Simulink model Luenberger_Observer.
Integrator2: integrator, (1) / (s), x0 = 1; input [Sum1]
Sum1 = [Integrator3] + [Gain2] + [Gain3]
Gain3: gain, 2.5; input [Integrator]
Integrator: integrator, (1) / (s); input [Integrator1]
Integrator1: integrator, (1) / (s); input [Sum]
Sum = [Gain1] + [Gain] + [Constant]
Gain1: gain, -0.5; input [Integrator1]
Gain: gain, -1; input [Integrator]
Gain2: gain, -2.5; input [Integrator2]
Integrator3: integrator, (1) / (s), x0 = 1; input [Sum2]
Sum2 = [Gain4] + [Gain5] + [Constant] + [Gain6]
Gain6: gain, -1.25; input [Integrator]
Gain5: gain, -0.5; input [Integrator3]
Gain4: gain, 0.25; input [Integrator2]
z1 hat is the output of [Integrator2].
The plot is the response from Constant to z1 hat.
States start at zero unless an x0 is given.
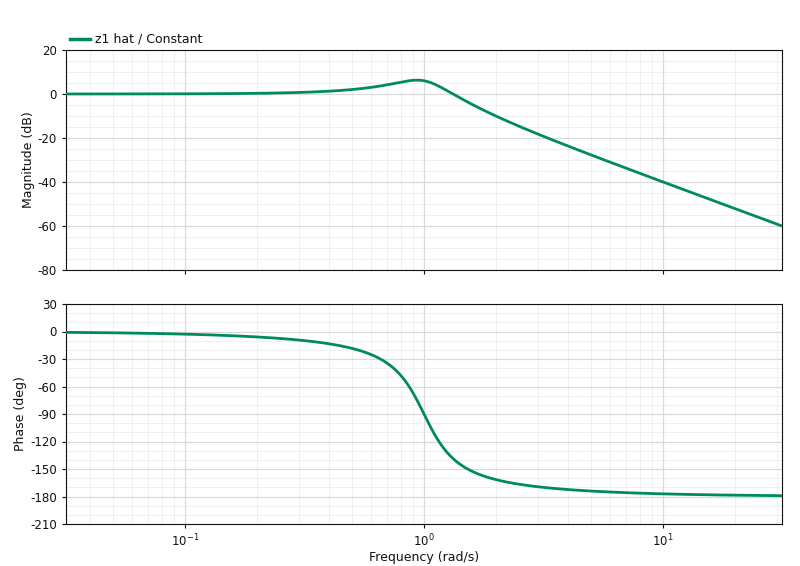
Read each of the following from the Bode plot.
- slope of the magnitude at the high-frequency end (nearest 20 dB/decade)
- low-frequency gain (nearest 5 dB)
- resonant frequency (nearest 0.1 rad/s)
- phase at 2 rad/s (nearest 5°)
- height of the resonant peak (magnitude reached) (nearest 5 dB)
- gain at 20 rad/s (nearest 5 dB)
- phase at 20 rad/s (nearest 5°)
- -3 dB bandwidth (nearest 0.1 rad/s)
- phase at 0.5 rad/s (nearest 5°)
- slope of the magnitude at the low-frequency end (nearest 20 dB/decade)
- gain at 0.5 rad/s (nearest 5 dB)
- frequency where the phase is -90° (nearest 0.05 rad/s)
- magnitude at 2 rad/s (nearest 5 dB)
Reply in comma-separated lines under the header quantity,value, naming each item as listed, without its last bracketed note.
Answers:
quantity,value
slope of the magnitude at the high-frequency end,-40 dB/decade
low-frequency gain,0 dB
resonant frequency,0.9 rad/s
phase at 2 rad/s,-160°
height of the resonant peak (magnitude reached),5 dB
gain at 20 rad/s,-50 dB
phase at 20 rad/s,-180°
-3 dB bandwidth,1.5 rad/s
phase at 0.5 rad/s,-20°
slope of the magnitude at the low-frequency end,0 dB/decade
gain at 0.5 rad/s,0 dB
frequency where the phase is -90°,1.00 rad/s
magnitude at 2 rad/s,-10 dB
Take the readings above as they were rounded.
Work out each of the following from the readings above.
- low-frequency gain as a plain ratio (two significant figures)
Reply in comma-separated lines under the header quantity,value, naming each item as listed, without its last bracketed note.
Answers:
quantity,value
low-frequency gain as a plain ratio,1.0
